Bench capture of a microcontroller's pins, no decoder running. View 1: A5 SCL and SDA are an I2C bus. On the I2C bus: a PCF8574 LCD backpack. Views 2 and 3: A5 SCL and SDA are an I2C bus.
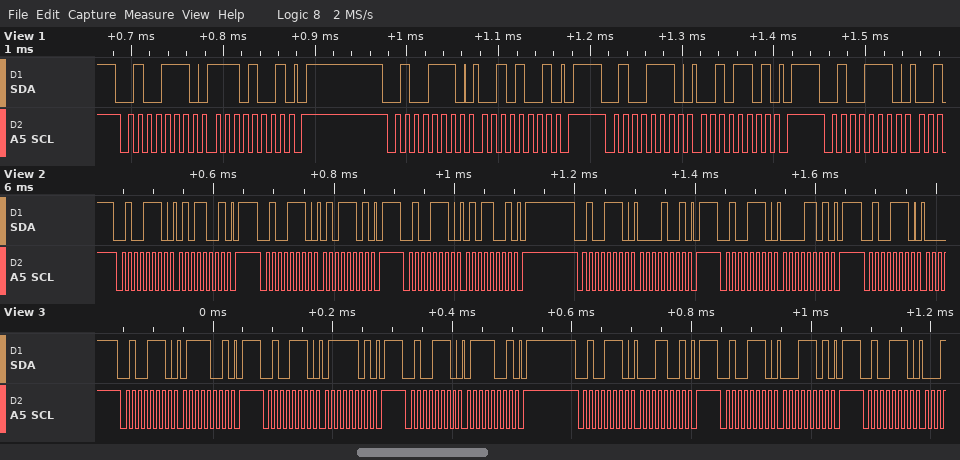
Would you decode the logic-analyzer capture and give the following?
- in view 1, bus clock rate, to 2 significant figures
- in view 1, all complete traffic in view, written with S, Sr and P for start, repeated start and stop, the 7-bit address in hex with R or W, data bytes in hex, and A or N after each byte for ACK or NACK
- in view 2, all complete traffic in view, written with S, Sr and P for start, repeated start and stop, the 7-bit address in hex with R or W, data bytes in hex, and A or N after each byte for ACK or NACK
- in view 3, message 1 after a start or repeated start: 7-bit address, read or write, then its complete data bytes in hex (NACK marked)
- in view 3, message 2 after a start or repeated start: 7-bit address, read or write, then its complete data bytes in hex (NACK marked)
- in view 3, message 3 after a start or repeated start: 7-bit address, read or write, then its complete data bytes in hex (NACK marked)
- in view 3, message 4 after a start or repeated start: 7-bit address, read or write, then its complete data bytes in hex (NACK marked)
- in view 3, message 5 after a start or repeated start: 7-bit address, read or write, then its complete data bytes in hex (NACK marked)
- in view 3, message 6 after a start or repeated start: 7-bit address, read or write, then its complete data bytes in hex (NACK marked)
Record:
100 kHz
S 27W A E9 A P S 27W A 29 A P S 27W A 2D A P S 27W A
S 27W A 59 A P S 27W A 5D A P S 27W A 59 A P S 27W A 09 A P S 27W A 0D A P S 27W A
0x27 write: 79
0x27 write: 7D
0x27 write: 79
0x27 write: 19
0x27 write: 1D
0x27 write
